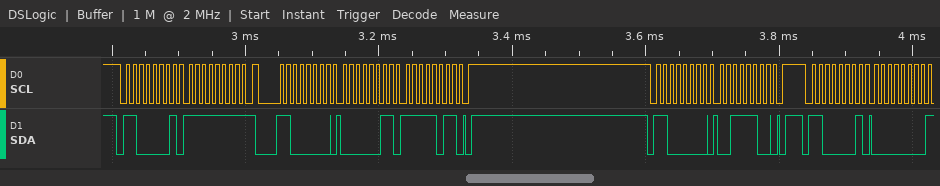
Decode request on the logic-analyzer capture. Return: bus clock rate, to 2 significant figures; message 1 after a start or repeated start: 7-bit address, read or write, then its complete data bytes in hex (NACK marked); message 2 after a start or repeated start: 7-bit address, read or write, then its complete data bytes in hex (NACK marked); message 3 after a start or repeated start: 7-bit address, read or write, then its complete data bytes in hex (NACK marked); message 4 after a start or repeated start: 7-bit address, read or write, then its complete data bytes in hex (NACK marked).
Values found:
100 kHz
0x60 read: FF NACK
0x60 write: 03 FB
0x60 write: 3C
0x60 read: 00 NACK
